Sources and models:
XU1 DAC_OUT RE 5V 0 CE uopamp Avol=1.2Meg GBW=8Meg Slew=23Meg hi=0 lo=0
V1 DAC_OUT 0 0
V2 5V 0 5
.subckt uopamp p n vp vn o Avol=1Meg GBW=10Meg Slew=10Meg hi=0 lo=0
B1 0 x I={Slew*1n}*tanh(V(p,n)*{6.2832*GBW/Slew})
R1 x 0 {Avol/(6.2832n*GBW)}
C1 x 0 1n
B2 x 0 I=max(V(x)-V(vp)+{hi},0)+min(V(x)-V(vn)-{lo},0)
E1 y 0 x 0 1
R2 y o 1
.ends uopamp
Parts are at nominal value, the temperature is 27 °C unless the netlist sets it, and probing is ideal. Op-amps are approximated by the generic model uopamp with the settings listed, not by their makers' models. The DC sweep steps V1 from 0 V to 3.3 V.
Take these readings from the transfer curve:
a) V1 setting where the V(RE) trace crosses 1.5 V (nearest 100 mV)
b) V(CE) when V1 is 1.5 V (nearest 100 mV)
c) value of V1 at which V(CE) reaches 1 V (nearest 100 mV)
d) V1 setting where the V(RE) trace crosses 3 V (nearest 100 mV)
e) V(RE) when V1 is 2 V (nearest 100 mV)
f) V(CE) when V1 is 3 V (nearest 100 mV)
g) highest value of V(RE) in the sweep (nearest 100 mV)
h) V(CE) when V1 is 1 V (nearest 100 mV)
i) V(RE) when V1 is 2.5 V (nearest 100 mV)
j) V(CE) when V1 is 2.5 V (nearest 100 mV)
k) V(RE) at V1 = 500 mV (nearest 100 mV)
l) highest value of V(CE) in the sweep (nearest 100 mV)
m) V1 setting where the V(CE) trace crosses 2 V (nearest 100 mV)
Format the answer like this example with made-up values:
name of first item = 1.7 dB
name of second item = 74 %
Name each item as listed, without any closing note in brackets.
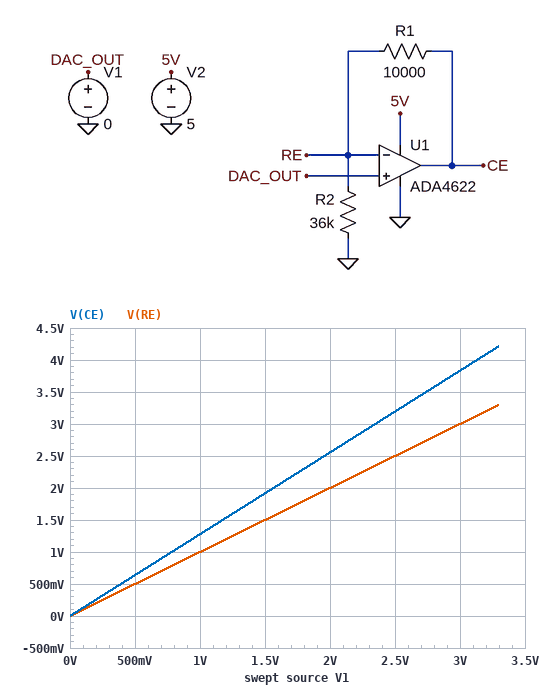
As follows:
V1 setting where the V(RE) trace crosses 1.5 V = 1.5 V
V(CE) when V1 is 1.5 V = 1.9 V
value of V1 at which V(CE) reaches 1 V = 800 mV
V1 setting where the V(RE) trace crosses 3 V = 3.0 V
V(RE) when V1 is 2 V = 2.0 V
V(CE) when V1 is 3 V = 3.8 V
highest value of V(RE) in the sweep = 3.3 V
V(CE) when V1 is 1 V = 1.3 V
V(RE) when V1 is 2.5 V = 2.5 V
V(CE) when V1 is 2.5 V = 3.2 V
V(RE) at V1 = 500 mV = 500 mV
highest value of V(CE) in the sweep = 4.2 V
V1 setting where the V(CE) trace crosses 2 V = 1.6 V
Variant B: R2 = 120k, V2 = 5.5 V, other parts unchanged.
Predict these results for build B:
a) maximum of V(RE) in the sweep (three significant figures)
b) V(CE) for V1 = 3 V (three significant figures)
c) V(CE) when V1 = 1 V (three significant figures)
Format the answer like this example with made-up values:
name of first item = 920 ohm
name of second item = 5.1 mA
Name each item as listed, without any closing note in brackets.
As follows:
maximum of V(RE) in the sweep = 3.30 V
V(CE) for V1 = 3 V = 3.25 V
V(CE) when V1 = 1 V = 1.08 V
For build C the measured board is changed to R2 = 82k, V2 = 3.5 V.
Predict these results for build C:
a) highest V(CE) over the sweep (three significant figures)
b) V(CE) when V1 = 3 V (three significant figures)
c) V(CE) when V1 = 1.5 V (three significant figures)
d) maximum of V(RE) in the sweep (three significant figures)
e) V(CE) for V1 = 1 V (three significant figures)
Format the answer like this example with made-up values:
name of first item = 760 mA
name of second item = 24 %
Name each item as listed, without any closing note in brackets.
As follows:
highest V(CE) over the sweep = 3.51 V
V(CE) when V1 = 3 V = 3.37 V
V(CE) when V1 = 1.5 V = 1.68 V
maximum of V(RE) in the sweep = 3.13 V
V(CE) for V1 = 1 V = 1.12 V
